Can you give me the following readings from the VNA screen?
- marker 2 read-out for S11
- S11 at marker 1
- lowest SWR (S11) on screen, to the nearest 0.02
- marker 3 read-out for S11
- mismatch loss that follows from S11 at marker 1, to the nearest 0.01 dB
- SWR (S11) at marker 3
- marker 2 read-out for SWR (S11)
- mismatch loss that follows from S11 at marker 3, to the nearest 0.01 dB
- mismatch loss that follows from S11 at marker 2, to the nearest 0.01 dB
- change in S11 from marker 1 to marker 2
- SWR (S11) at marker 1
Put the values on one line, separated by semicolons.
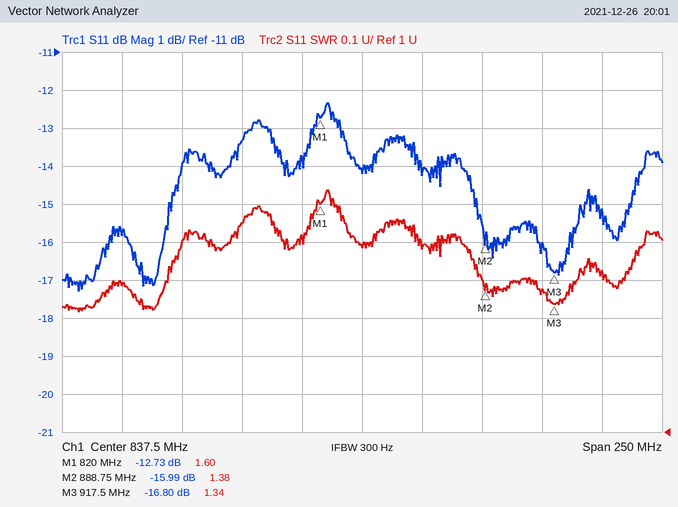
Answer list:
-15.99 dB; -12.73 dB; 1.32; -16.80 dB; 0.24 dB; 1.34; 1.38; 0.09 dB; 0.11 dB; -3.26 dB; 1.60
